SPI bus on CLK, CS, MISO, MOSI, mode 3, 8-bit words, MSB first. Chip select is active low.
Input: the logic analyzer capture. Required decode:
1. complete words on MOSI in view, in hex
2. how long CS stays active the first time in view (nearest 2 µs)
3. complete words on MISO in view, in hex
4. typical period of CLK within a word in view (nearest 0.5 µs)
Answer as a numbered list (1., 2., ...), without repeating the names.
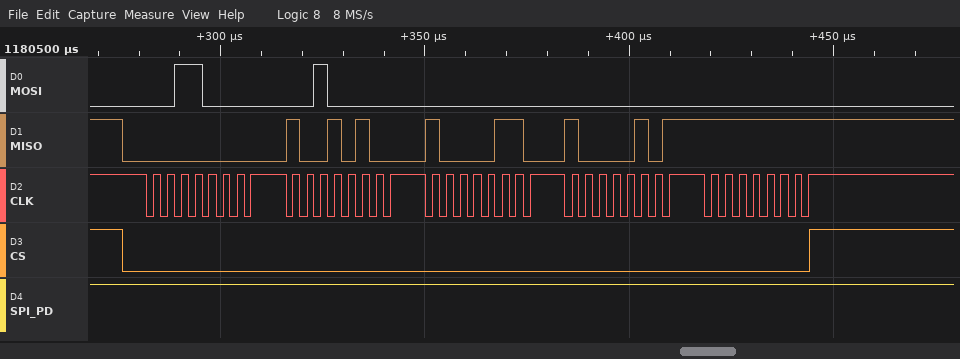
1. 30, 20, 00, 00, 00
2. 168 µs
3. 00, 94, 86, 85, FF
4. 3.5 µs
